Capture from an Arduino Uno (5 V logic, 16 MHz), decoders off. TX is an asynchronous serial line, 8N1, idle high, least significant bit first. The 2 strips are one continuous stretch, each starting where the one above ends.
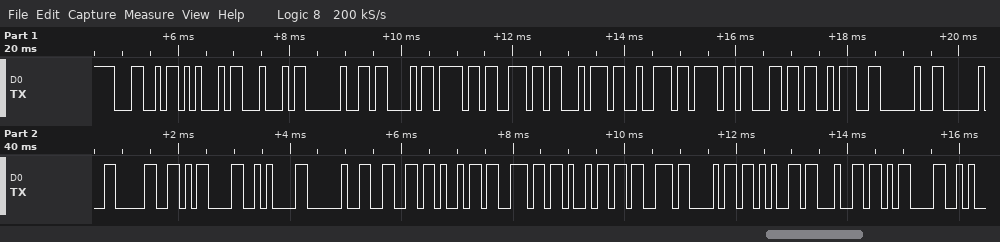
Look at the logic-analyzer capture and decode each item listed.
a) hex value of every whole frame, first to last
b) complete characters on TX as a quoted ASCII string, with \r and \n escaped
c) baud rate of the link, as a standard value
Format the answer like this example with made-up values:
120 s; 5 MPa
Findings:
4C 45 44 20 43 6F 6E 74 72 6F 6C 3A 20 20 30 0D 0A 20 66 69 6E 69 73 68 65 64 0D; "LED Control:  0\r\n finished\r"; 9600 baud
